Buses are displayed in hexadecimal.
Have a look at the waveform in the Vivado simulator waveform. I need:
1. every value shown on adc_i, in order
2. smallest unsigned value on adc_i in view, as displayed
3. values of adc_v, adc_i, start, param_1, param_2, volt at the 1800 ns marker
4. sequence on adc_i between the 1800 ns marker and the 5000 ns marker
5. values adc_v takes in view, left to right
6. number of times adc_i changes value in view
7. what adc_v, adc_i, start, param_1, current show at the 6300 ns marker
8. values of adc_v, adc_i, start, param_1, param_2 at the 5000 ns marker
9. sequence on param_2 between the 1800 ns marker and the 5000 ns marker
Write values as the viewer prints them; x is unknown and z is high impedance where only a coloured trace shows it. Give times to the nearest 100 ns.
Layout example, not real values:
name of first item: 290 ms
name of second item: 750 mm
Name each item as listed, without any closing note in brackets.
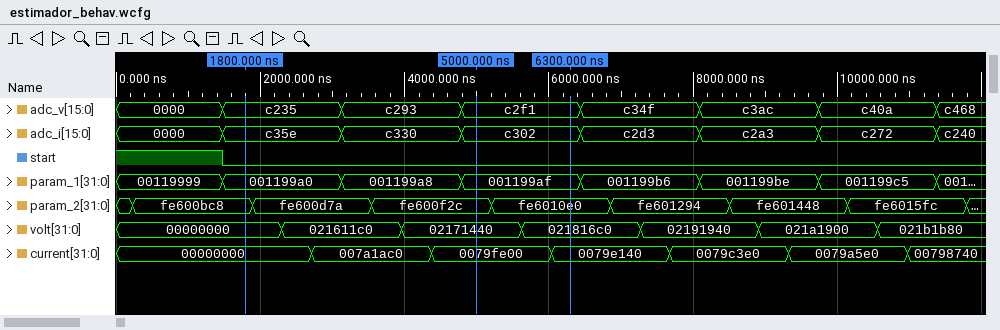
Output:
every value shown on adc_i, in order: 0000, c35e, c330, c302, c2d3, c2a3, c272, c240
smallest unsigned value on adc_i in view, as displayed: 0000
values of adc_v, adc_i, start, param_1, param_2, volt at the 1800 ns marker: adc_v=c235, adc_i=c35e, start=0, param_1=001199a0, param_2=fe600bc8, volt=00000000
sequence on adc_i between the 1800 ns marker and the 5000 ns marker: c35e, c330, c302
values adc_v takes in view, left to right: 0000, c235, c293, c2f1, c34f, c3ac, c40a, c468
number of times adc_i changes value in view: 7
what adc_v, adc_i, start, param_1, current show at the 6300 ns marker: adc_v=c2f1, adc_i=c302, start=0, param_1=001199af, current=0079e140
values of adc_v, adc_i, start, param_1, param_2 at the 5000 ns marker: adc_v=c2f1, adc_i=c302, start=0, param_1=001199af, param_2=fe600f2c
sequence on param_2 between the 1800 ns marker and the 5000 ns marker: fe600bc8, fe600d7a, fe600f2c
